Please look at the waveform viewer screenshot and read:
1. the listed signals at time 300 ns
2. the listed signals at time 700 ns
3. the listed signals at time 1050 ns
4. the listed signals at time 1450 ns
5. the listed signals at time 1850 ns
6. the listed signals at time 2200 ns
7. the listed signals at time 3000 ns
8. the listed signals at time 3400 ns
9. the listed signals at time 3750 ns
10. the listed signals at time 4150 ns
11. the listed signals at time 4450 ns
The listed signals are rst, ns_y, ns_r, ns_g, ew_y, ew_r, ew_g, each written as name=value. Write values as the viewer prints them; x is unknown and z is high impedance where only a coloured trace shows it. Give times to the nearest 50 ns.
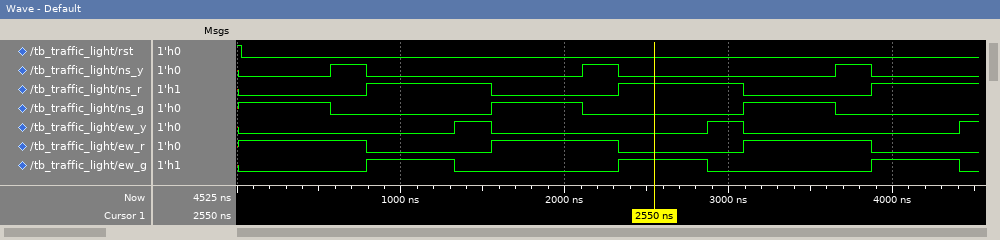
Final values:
rst=0, ns_y=0, ns_r=0, ns_g=1, ew_y=0, ew_r=1, ew_g=0
rst=0, ns_y=1, ns_r=0, ns_g=0, ew_y=0, ew_r=1, ew_g=0
rst=0, ns_y=0, ns_r=1, ns_g=0, ew_y=0, ew_r=0, ew_g=1
rst=0, ns_y=0, ns_r=1, ns_g=0, ew_y=1, ew_r=0, ew_g=0
rst=0, ns_y=0, ns_r=0, ns_g=1, ew_y=0, ew_r=1, ew_g=0
rst=0, ns_y=1, ns_r=0, ns_g=0, ew_y=0, ew_r=1, ew_g=0
rst=0, ns_y=0, ns_r=1, ns_g=0, ew_y=1, ew_r=0, ew_g=0
rst=0, ns_y=0, ns_r=0, ns_g=1, ew_y=0, ew_r=1, ew_g=0
rst=0, ns_y=1, ns_r=0, ns_g=0, ew_y=0, ew_r=1, ew_g=0
rst=0, ns_y=0, ns_r=1, ns_g=0, ew_y=0, ew_r=0, ew_g=1
rst=0, ns_y=0, ns_r=1, ns_g=0, ew_y=1, ew_r=0, ew_g=0
